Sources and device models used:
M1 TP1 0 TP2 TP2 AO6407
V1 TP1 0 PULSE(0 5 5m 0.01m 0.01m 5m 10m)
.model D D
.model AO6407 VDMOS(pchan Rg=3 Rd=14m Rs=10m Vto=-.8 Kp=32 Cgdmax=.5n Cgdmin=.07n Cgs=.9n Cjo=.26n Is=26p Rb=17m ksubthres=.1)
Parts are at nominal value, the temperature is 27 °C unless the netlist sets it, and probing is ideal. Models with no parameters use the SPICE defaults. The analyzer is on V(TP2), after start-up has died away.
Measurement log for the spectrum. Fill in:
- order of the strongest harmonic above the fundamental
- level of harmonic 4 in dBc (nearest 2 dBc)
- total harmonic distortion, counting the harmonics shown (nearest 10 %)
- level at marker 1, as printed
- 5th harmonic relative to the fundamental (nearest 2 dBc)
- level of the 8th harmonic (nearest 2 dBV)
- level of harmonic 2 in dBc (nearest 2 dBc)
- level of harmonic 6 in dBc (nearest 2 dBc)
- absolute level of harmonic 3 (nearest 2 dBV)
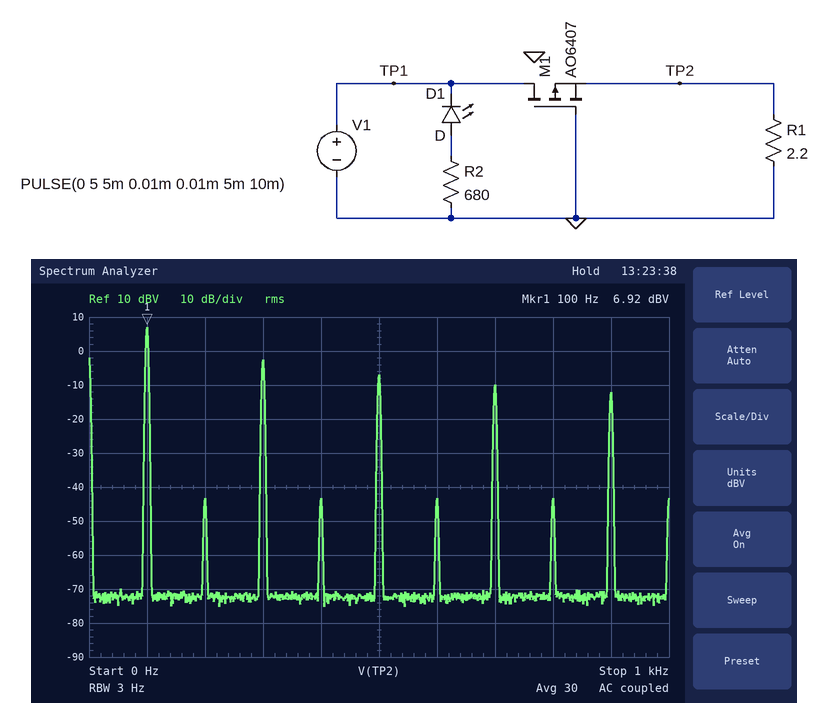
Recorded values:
3
-50 dBc
40 %
6.92 dBV
-14 dBc
-44 dBV
-50 dBc
-50 dBc
-2 dBV
